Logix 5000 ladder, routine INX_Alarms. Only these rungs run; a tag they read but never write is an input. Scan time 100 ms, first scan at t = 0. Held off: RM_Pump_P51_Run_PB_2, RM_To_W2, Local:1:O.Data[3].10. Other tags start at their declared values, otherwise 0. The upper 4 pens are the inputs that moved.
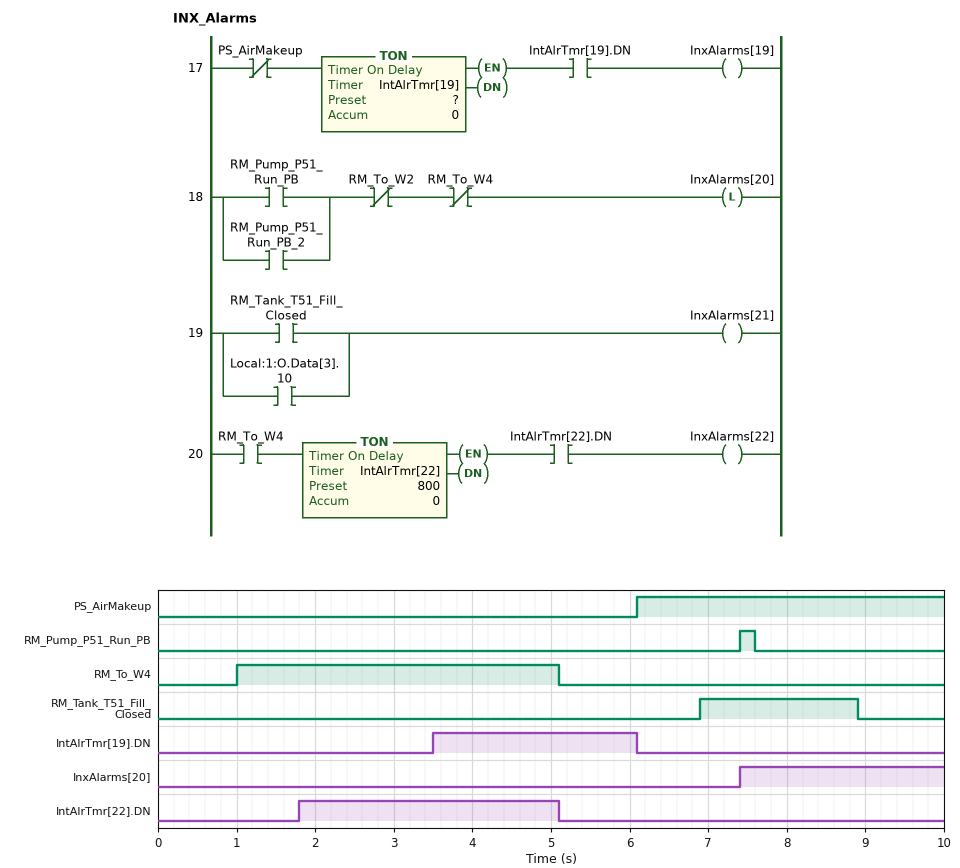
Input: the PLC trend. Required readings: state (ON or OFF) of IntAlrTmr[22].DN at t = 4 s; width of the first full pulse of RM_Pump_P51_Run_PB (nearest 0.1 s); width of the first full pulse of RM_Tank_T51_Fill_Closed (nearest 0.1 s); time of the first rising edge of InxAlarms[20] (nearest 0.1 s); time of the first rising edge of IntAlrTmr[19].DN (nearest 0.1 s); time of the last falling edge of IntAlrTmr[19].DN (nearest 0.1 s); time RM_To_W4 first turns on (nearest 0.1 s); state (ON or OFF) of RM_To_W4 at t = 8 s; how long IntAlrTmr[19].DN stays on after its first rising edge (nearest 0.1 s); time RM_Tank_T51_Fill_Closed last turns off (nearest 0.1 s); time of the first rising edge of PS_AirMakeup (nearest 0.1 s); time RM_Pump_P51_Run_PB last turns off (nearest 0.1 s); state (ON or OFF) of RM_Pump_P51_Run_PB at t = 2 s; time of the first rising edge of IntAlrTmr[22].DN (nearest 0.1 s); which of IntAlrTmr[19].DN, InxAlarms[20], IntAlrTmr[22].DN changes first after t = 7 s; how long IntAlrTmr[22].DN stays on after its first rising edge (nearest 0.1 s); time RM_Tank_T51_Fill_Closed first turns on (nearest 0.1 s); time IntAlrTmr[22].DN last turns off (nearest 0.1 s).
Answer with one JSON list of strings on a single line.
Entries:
["ON", "0.2 s", "2.0 s", "7.4 s", "3.5 s", "6.1 s", "1.0 s", "OFF", "2.6 s", "8.9 s", "6.1 s", "7.6 s", "OFF", "1.8 s", "InxAlarms[20]", "3.3 s", "6.9 s", "5.1 s"]
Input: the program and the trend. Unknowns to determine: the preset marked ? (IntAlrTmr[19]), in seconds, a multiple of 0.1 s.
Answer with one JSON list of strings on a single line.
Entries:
["3.5 s"]
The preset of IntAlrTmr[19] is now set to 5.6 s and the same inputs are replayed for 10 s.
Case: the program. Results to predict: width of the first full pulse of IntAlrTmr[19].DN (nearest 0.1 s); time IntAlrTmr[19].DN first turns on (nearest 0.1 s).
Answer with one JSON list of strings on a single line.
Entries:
["0.5 s", "5.6 s"]
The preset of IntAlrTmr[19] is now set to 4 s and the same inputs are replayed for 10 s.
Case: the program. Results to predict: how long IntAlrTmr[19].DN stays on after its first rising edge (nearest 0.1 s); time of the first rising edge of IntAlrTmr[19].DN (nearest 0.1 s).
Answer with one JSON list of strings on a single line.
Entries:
["2.1 s", "4.0 s"]
